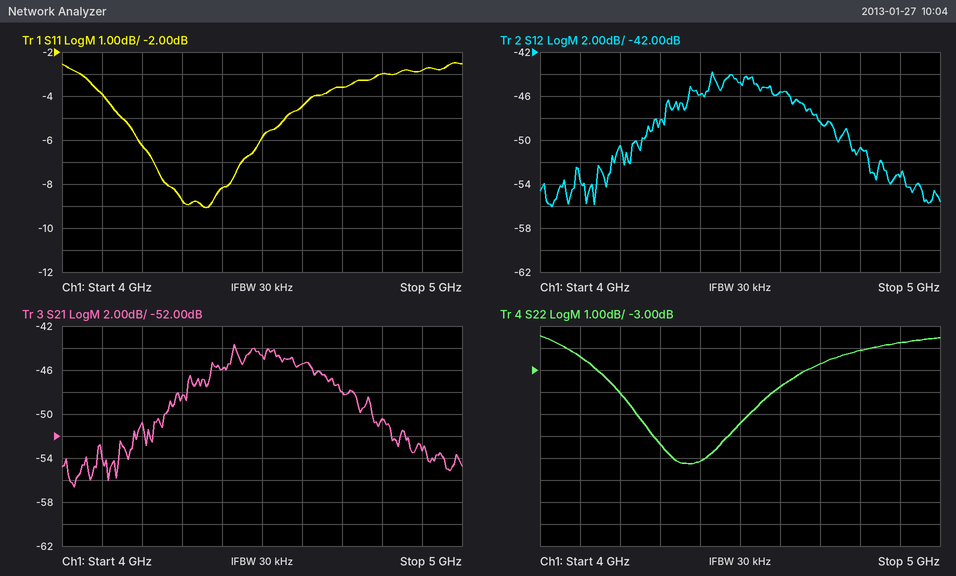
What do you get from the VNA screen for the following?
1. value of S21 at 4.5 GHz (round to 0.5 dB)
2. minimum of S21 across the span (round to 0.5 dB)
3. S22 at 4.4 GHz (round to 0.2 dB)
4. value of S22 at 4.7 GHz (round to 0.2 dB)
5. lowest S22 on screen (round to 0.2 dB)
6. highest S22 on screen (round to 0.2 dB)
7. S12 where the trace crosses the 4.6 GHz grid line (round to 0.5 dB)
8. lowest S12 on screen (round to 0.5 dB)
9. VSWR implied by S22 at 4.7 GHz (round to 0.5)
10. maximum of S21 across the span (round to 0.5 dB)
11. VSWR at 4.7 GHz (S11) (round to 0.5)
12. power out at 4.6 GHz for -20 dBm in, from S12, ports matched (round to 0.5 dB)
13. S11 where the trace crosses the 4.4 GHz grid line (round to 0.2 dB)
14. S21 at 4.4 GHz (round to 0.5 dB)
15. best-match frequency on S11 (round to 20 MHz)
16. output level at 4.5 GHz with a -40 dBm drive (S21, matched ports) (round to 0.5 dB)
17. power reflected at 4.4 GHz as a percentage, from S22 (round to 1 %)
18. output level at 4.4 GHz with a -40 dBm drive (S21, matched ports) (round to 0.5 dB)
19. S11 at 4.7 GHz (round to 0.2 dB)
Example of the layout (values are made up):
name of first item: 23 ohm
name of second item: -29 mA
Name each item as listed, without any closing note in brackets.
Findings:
value of S21 at 4.5 GHz: -44.5 dB
minimum of S21 across the span: -56.5 dB
S22 at 4.4 GHz: -7.2 dB
value of S22 at 4.7 GHz: -2.8 dB
lowest S22 on screen: -7.2 dB
highest S22 on screen: -1.4 dB
S12 where the trace crosses the 4.6 GHz grid line: -45.5 dB
lowest S12 on screen: -56.0 dB
VSWR implied by S22 at 4.7 GHz: 6.5
maximum of S21 across the span: -43.5 dB
VSWR at 4.7 GHz (S11): 5.0
power out at 4.6 GHz for -20 dBm in, from S12, ports matched: -65.5 dBm
S11 where the trace crosses the 4.4 GHz grid line: -8.2 dB
S21 at 4.4 GHz: -46.0 dB
best-match frequency on S11: 4.36 GHz
output level at 4.5 GHz with a -40 dBm drive (S21, matched ports): -84.5 dBm
power reflected at 4.4 GHz as a percentage, from S22: 19 %
output level at 4.4 GHz with a -40 dBm drive (S21, matched ports): -86.0 dBm
S11 at 4.7 GHz: -3.6 dB
